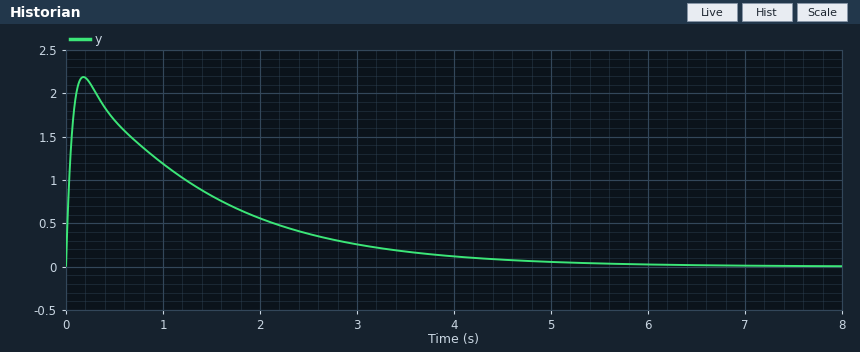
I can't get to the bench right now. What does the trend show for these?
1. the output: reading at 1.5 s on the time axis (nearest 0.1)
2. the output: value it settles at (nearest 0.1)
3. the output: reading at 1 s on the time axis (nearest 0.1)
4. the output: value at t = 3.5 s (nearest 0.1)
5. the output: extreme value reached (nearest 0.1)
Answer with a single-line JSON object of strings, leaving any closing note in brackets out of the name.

{"the output: reading at 1.5 s on the time axis": "0.8", "the output: value it settles at": "0.0", "the output: reading at 1 s on the time axis": "1.2", "the output: value at t = 3.5 s": "0.2", "the output: extreme value reached": "2.2"}
